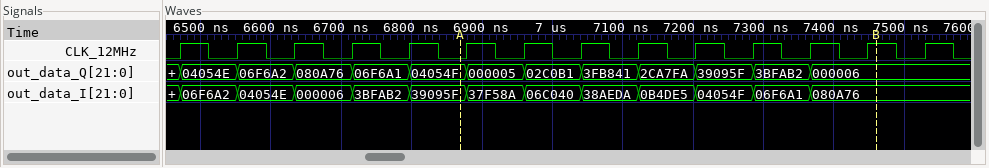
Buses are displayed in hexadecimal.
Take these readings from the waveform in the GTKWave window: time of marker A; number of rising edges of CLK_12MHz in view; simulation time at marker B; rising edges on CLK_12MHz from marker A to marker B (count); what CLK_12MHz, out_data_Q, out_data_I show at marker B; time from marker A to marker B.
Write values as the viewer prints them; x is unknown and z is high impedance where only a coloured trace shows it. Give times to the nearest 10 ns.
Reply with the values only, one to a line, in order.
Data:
6870 ns
14
7460 ns
8
CLK_12MHz=1, out_data_Q=000006, out_data_I=080A76
590 ns
